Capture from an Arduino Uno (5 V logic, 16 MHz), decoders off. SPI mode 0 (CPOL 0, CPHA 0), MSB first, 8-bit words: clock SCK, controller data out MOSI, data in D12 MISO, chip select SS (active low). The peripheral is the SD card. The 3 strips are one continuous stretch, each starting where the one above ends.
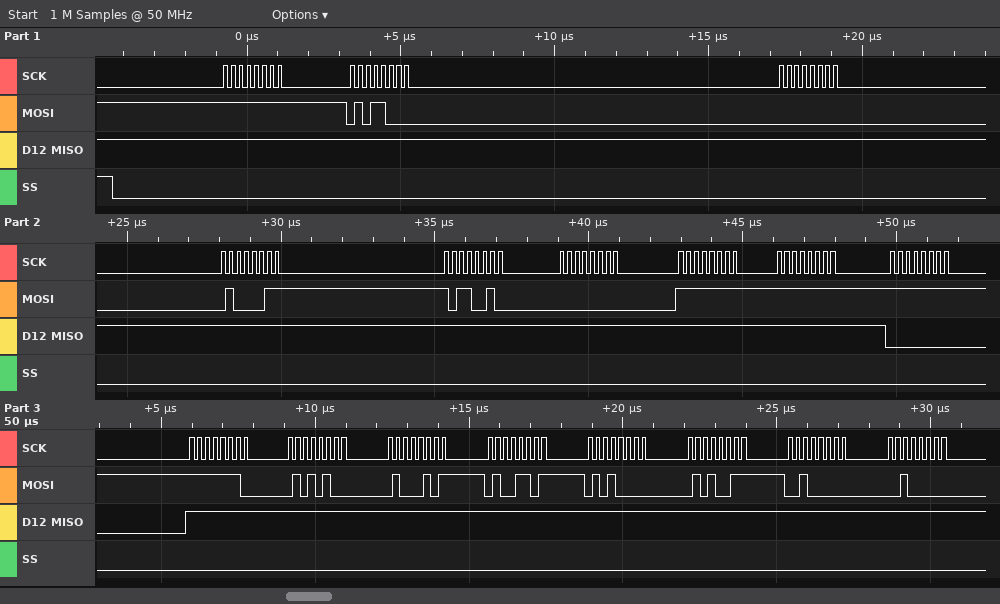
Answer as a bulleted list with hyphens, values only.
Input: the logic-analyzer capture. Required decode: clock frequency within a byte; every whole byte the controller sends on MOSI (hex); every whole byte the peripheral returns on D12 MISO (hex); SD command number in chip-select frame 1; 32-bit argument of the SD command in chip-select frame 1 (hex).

- 4 MHz
- FF 58 00 43 B2 00 FF FF FF FE 54 45 4D 50 53 20 20
- FF FF FF FF FF FF FF FF 00 FF FF FF FF FF FF FF FF
- CMD24
- 0x0043B200
